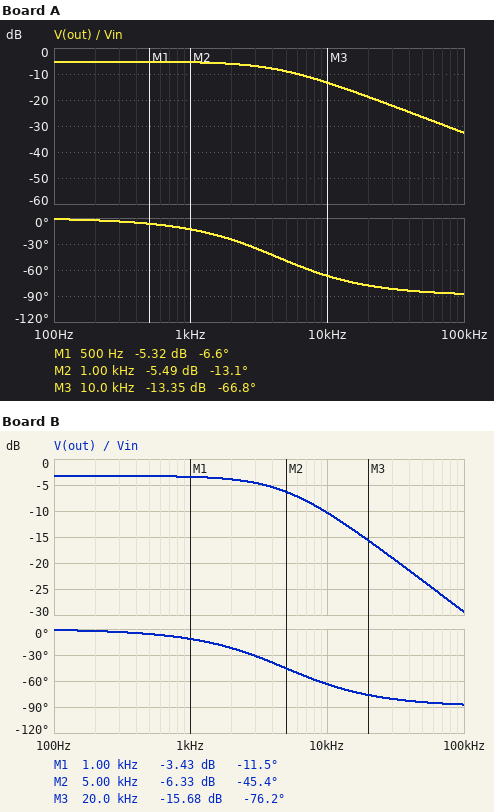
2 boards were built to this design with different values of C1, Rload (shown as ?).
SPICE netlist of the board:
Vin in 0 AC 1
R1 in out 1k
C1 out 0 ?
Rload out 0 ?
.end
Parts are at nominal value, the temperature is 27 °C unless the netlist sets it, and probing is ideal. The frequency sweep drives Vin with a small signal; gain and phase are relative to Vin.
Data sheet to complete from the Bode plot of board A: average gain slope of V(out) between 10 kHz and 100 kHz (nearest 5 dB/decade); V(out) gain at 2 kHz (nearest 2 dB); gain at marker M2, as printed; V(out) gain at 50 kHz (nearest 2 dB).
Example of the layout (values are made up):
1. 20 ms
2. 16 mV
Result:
1. -20 dB/decade
2. -6 dB
3. -5.49 dB
4. -26 dB
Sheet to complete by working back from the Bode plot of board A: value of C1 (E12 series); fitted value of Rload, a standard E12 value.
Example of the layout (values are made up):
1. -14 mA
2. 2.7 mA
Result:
1. 68 nF
2. 1.2 kΩ
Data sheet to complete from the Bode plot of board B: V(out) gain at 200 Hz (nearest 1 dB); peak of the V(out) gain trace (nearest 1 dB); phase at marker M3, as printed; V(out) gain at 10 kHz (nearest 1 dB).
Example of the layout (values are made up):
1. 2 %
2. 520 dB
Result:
1. -3 dB
2. -3 dB
3. -76.2 deg
4. -10 dB
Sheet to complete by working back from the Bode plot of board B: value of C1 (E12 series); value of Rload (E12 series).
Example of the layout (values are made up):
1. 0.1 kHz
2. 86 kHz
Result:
1. 47 nF
2. 2.2 kΩ
